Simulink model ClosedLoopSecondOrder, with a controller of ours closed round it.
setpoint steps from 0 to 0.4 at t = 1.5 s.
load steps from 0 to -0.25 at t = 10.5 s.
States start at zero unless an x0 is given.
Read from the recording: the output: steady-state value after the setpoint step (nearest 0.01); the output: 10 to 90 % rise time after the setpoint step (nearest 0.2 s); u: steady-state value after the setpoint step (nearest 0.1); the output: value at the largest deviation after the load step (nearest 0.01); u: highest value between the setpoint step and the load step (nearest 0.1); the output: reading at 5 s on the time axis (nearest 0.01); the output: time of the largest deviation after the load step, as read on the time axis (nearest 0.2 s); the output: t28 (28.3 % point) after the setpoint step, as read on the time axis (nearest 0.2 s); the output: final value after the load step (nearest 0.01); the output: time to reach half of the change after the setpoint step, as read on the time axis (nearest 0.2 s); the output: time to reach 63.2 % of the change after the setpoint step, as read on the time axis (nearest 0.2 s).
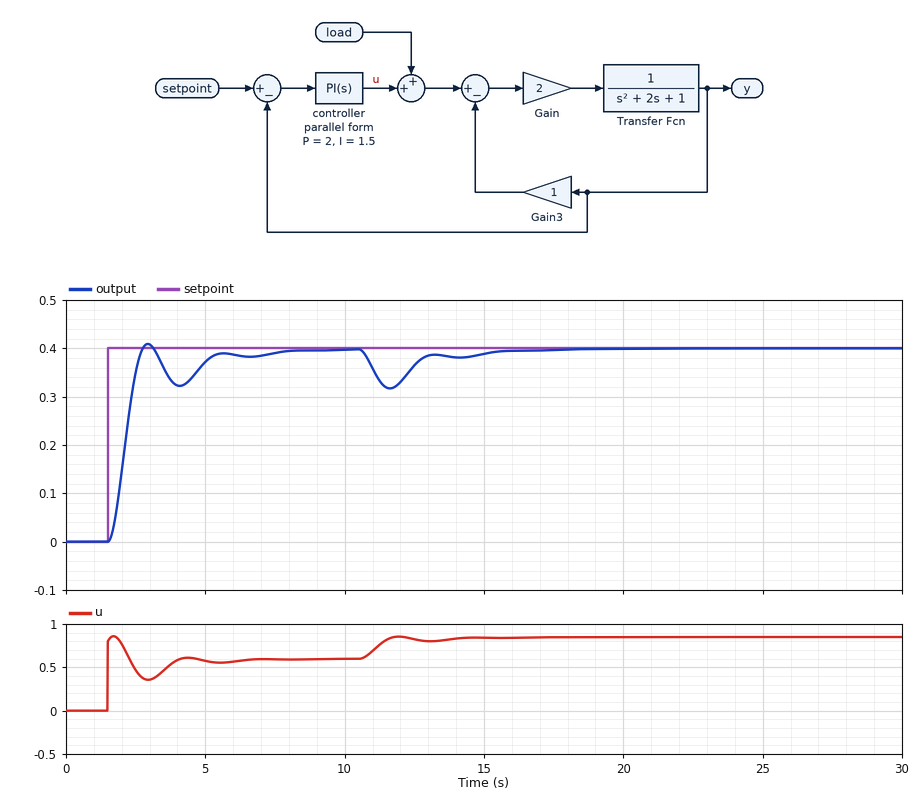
0.40
0.8 s
0.6
0.32
0.9
0.37
11.6 s
2.0 s
0.40
2.2 s
2.2 s
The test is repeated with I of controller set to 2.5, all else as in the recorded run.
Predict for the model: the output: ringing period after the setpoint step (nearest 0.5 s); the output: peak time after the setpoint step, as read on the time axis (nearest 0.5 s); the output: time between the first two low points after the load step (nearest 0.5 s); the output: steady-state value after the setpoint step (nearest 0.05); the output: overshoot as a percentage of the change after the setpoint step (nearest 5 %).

2.5 s
3.0 s
2.5 s
0.40
20 %
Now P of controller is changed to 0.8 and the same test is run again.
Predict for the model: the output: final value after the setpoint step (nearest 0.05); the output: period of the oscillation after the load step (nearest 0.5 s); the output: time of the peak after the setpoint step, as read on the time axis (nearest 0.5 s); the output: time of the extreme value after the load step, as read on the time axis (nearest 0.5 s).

0.40
3.5 s
3.5 s
12.0 s
